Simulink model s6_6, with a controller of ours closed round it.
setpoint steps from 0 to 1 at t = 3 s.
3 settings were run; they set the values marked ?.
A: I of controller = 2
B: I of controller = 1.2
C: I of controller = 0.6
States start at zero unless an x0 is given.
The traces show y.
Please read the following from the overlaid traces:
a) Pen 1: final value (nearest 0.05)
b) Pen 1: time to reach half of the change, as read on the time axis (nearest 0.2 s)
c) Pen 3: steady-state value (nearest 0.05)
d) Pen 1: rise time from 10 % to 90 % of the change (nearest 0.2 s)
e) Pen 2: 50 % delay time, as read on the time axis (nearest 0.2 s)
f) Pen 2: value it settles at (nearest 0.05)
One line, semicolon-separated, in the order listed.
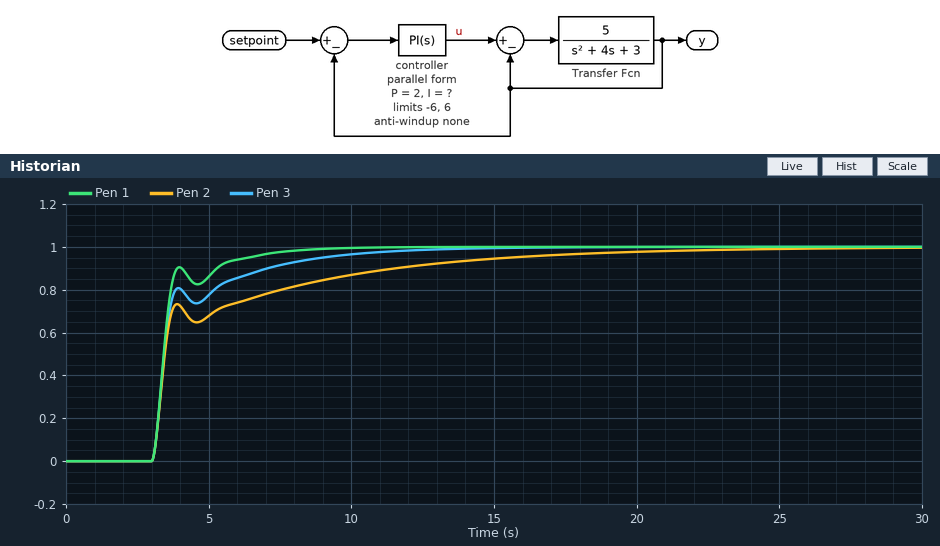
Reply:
1.00; 3.4 s; 1.00; 0.8 s; 3.4 s; 1.00
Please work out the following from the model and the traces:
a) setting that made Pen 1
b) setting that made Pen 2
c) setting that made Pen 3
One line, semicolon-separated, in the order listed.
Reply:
A; C; B
